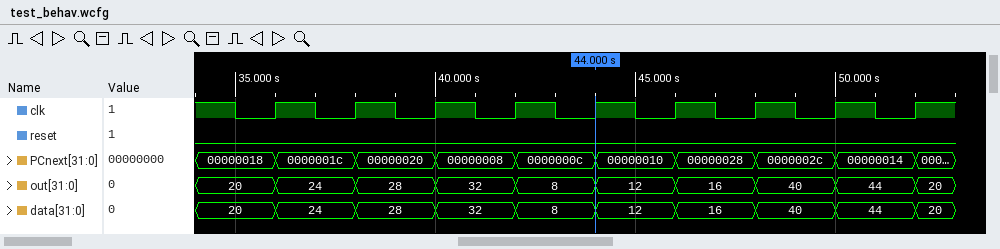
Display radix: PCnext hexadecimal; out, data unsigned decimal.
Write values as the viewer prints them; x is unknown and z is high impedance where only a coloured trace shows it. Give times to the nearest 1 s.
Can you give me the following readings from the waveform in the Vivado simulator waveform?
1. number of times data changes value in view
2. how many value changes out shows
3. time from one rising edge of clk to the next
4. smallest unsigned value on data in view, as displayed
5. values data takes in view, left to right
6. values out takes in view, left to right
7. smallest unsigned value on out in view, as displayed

9
9
2 s
8
20, 24, 28, 32, 8, 12, 16, 40, 44, 20
20, 24, 28, 32, 8, 12, 16, 40, 44, 20
8
